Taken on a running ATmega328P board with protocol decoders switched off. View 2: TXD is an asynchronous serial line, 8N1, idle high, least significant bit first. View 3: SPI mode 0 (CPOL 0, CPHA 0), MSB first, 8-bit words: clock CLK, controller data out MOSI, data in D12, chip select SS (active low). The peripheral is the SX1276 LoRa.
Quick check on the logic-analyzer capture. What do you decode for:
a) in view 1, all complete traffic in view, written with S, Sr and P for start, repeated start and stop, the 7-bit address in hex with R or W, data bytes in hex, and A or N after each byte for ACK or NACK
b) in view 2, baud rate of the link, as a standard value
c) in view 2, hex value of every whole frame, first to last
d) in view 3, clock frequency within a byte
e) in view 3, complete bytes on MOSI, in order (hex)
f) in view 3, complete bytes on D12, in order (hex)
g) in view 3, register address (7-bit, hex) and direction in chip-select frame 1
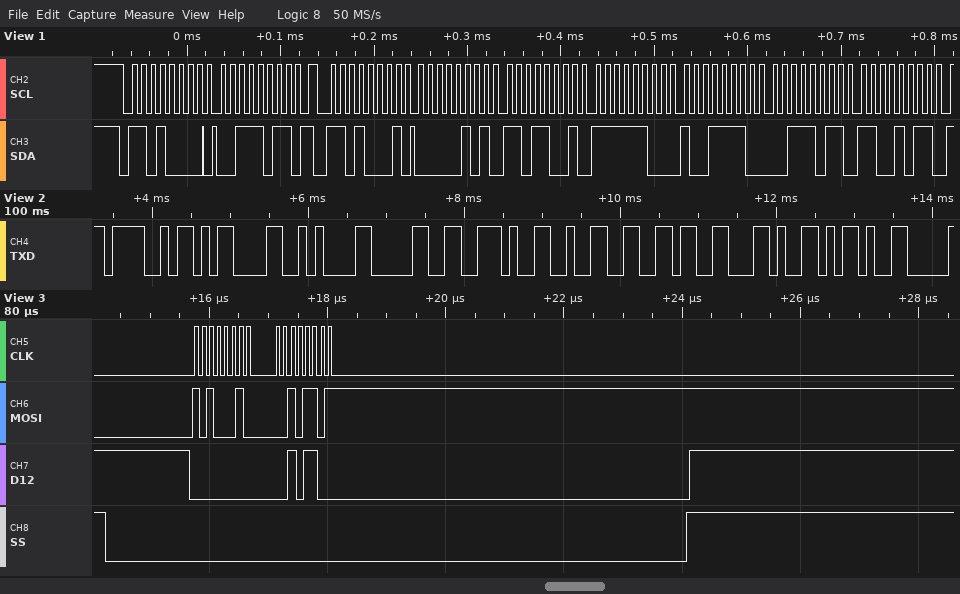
S 68W A 3B A Sr 68R A 05 A D9 A FC A 9E A 3B A CB A
9600 baud
4F 0D 0A 30 2E 32 36 2C 2D
8 MHz
0xA2 0x2D
0x00 0x2C
0x22 write
